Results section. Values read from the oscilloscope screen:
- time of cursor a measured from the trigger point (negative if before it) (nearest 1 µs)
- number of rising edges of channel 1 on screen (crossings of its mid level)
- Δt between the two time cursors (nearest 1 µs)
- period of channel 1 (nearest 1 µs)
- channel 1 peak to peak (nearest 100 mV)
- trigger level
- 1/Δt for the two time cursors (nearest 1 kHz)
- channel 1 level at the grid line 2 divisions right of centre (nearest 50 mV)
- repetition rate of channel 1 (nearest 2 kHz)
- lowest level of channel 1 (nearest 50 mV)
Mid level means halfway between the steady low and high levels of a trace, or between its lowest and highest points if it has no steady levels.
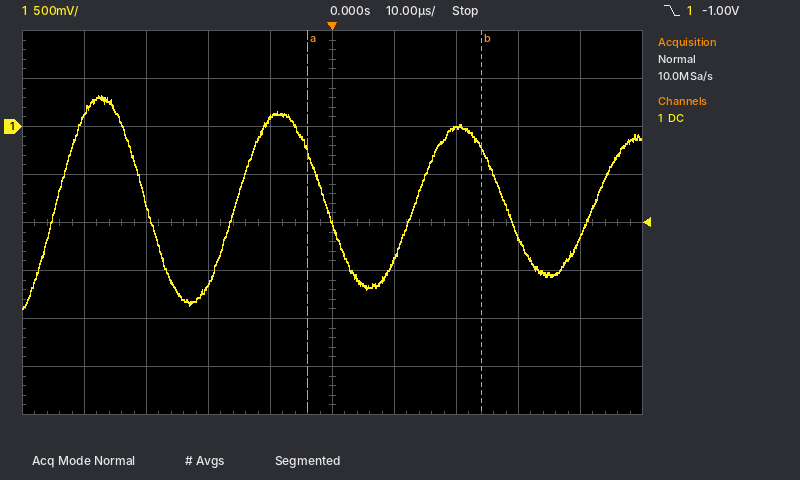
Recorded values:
-4 µs
4
28 µs
29 µs
2.20 V
-1.00 V
36 kHz
0 mV
34 kHz
-1.90 V
